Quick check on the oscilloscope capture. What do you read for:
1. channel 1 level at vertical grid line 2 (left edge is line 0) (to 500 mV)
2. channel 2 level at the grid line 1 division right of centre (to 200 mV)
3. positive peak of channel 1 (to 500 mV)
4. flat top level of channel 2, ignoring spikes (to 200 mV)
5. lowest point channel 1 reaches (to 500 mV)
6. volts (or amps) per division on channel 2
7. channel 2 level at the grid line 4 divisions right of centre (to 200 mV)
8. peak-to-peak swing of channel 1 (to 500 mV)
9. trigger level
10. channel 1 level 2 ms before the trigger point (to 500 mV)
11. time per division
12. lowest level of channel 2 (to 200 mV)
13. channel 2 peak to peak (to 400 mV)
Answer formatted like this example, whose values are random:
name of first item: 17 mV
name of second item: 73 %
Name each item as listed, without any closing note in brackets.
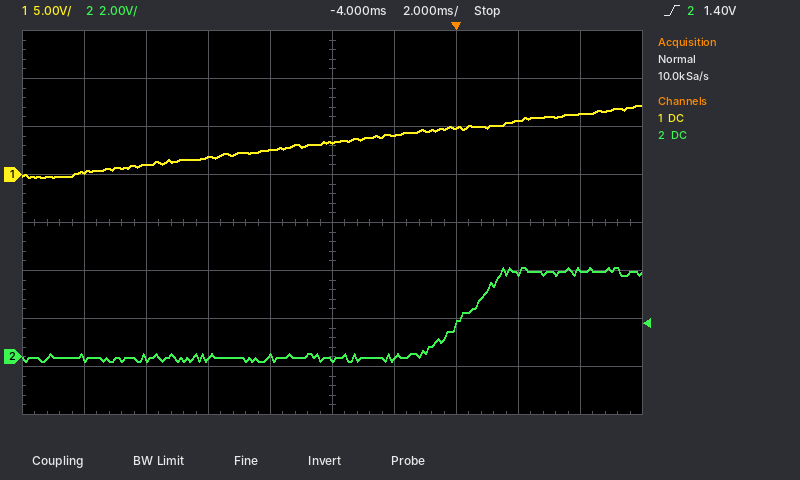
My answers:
channel 1 level at vertical grid line 2 (left edge is line 0): 1.0 V
channel 2 level at the grid line 1 division right of centre: 0.0 V
positive peak of channel 1: 7.0 V
flat top level of channel 2, ignoring spikes: 3.6 V
lowest point channel 1 reaches: -500 mV
volts (or amps) per division on channel 2: 2 V
channel 2 level at the grid line 4 divisions right of centre: 3.6 V
peak-to-peak swing of channel 1: 7.5 V
trigger level: 1.40 V
channel 1 level 2 ms before the trigger point: 4.0 V
time per division: 2 ms
lowest level of channel 2: -200 mV
channel 2 peak to peak: 4.0 V
